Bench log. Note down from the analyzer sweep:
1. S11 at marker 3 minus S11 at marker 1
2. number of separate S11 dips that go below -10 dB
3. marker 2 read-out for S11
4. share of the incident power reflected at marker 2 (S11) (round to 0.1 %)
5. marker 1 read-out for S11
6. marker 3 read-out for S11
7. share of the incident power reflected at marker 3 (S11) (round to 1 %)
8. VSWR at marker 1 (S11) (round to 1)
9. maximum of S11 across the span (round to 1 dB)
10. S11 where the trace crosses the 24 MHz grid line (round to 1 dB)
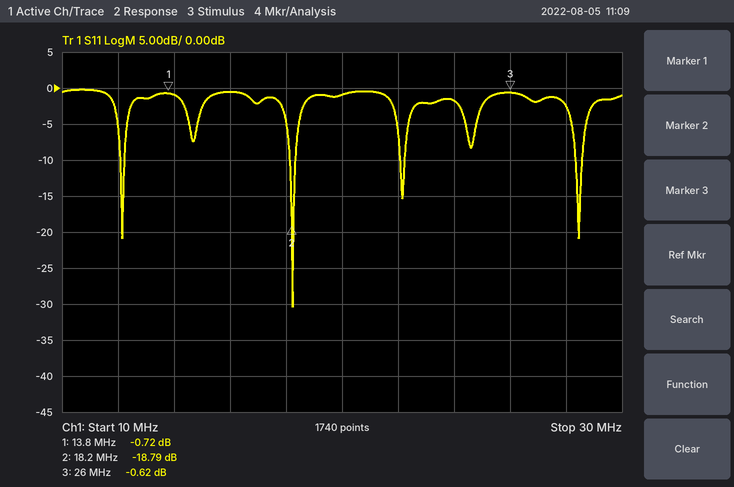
0.10 dB
4
-18.79 dB
1.3 %
-0.72 dB
-0.62 dB
87 %
24
0 dB
-2 dB
